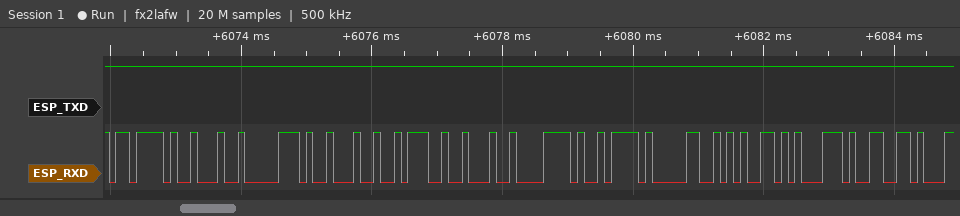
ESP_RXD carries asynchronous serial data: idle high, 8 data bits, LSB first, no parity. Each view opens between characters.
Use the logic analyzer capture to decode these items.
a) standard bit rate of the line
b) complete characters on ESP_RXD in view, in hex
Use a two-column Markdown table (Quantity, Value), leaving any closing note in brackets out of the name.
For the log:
| Quantity | Value |
|---|---|
| standard bit rate of the line | 9600 baud |
| complete characters on ESP_RXD in view, in hex | 7B, 22, 70, 22, 3A, 22, 78, 7A, 30, 65, 71, 66 |
